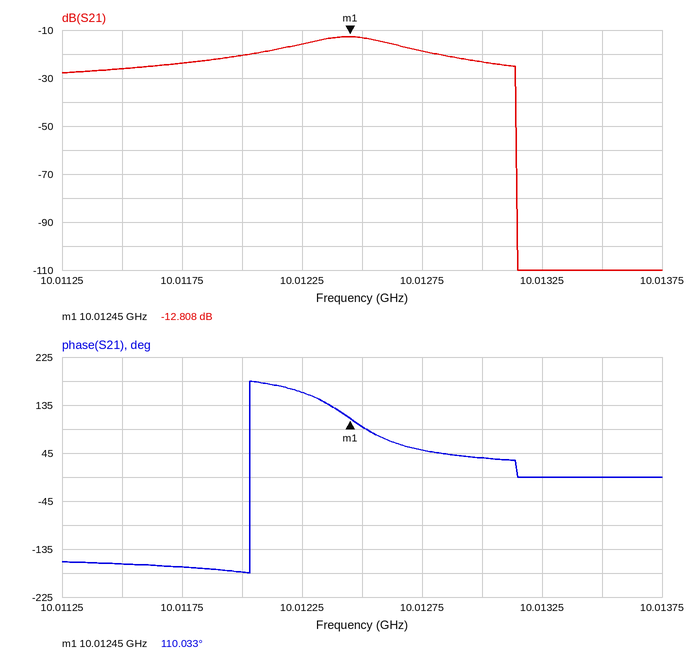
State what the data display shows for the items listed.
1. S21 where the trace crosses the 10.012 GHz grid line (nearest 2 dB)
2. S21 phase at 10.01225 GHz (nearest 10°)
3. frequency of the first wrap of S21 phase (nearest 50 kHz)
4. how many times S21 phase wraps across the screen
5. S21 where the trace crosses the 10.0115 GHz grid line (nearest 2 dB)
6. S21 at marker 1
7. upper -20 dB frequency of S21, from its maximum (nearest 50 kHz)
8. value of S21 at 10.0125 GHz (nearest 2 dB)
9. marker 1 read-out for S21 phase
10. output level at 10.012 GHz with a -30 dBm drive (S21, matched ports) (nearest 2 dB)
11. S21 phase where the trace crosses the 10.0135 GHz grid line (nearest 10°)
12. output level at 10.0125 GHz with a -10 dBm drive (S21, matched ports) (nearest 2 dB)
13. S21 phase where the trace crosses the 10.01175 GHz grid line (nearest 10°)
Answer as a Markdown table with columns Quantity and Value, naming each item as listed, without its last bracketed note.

| Quantity | Value |
|---|---|
| S21 where the trace crosses the 10.012 GHz grid line | -20 dB |
| S21 phase at 10.01225 GHz | 160° |
| frequency of the first wrap of S21 phase | 10.01205 GHz |
| how many times S21 phase wraps across the screen | 1 |
| S21 where the trace crosses the 10.0115 GHz grid line | -26 dB |
| S21 at marker 1 | -12.808 dB |
| upper -20 dB frequency of S21, from its maximum | 10.01315 GHz |
| value of S21 at 10.0125 GHz | -14 dB |
| marker 1 read-out for S21 phase | 110.033° |
| output level at 10.012 GHz with a -30 dBm drive (S21, matched ports) | -50 dBm |
| S21 phase where the trace crosses the 10.0135 GHz grid line | 0° |
| output level at 10.0125 GHz with a -10 dBm drive (S21, matched ports) | -24 dBm |
| S21 phase where the trace crosses the 10.01175 GHz grid line | -170° |
